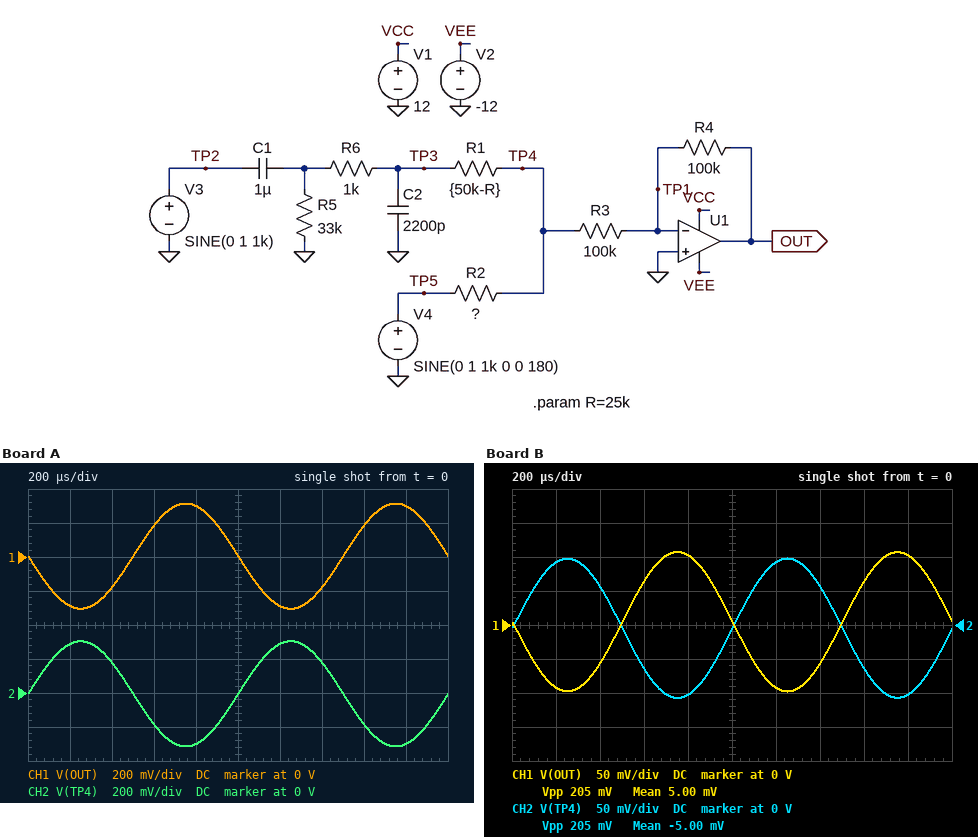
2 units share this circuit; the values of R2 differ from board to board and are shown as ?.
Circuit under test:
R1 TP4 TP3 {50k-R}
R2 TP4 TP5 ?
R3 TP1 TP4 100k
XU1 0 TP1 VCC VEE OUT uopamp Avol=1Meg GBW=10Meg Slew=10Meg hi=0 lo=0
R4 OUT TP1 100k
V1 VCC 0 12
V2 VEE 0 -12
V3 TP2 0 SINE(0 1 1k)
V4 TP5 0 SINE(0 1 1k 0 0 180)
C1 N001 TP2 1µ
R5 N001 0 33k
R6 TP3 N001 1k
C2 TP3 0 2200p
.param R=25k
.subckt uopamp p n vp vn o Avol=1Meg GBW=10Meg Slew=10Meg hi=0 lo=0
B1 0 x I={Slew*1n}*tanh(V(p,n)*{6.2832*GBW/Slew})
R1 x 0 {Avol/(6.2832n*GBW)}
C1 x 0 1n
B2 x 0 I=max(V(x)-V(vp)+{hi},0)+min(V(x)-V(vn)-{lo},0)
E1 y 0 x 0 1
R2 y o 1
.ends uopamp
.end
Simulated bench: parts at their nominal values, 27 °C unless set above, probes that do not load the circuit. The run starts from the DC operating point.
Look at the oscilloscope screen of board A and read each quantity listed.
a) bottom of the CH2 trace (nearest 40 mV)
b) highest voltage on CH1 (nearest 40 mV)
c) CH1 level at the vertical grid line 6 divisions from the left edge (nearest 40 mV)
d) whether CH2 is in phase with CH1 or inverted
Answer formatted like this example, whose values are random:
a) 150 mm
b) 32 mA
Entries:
a) -320 mV
b) 320 mV
c) -280 mV
d) inverted
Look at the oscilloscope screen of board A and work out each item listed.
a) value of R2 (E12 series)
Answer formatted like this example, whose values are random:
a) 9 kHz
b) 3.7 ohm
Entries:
a) 56 kΩ
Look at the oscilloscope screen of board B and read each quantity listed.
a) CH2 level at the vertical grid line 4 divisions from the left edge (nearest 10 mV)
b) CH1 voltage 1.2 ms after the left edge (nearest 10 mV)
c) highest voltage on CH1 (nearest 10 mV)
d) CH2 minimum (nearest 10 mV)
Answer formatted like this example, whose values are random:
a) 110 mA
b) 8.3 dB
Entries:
a) -100 mV
b) -90 mV
c) 110 mV
d) -110 mV
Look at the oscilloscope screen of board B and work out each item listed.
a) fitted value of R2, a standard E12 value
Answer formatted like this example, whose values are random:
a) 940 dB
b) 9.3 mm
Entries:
a) 33 kΩ
